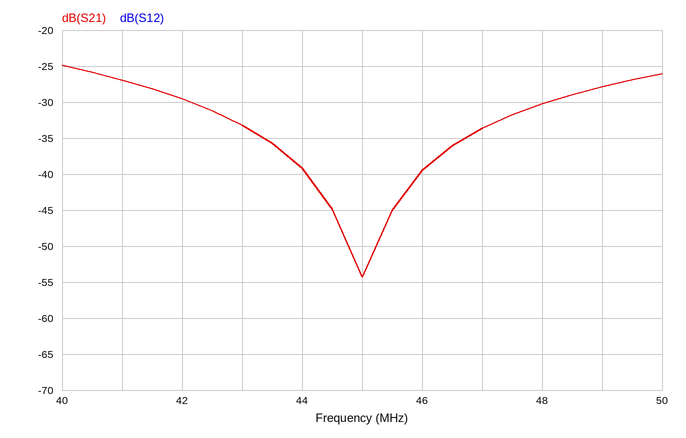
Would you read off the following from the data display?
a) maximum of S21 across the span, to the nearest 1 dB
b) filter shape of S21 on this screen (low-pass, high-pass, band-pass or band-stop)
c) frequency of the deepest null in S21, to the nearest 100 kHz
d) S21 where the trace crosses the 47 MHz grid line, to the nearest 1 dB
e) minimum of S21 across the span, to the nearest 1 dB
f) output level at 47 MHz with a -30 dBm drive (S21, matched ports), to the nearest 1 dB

-25 dB
band-stop
45.0 MHz
-34 dB
-54 dB
-64 dBm
